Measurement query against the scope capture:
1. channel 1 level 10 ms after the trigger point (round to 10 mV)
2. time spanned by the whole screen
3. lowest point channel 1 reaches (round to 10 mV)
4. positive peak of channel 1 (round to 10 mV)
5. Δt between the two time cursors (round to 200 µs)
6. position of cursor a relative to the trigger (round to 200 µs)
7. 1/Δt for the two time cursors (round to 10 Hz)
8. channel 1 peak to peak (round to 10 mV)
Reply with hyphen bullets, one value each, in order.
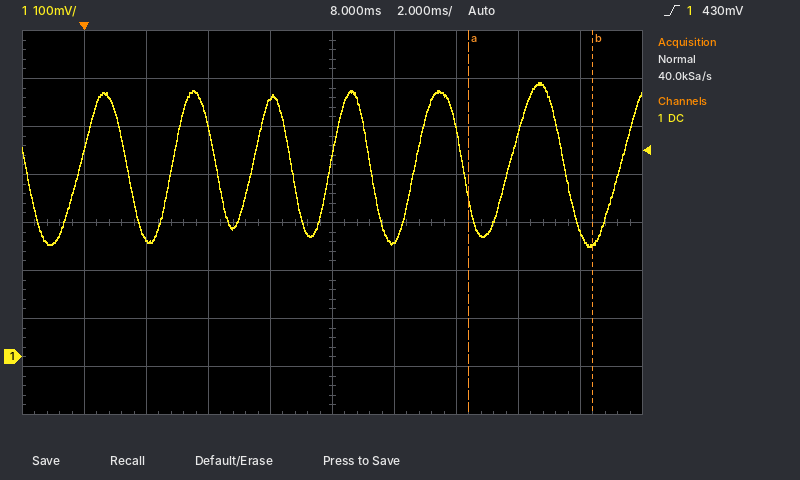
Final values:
- 240 mV
- 20 ms
- 230 mV
- 570 mV
- 4.0 ms
- +12.4 ms
- 250 Hz
- 340 mV
